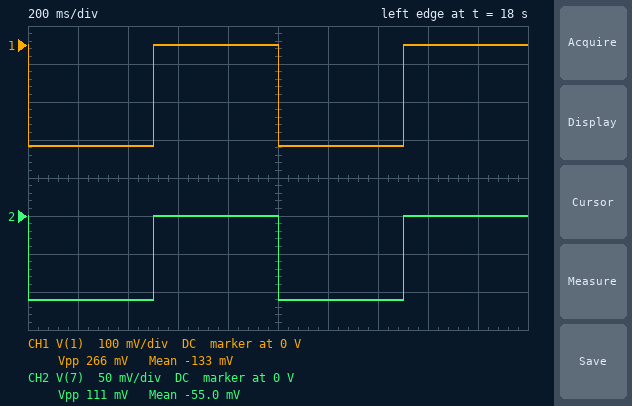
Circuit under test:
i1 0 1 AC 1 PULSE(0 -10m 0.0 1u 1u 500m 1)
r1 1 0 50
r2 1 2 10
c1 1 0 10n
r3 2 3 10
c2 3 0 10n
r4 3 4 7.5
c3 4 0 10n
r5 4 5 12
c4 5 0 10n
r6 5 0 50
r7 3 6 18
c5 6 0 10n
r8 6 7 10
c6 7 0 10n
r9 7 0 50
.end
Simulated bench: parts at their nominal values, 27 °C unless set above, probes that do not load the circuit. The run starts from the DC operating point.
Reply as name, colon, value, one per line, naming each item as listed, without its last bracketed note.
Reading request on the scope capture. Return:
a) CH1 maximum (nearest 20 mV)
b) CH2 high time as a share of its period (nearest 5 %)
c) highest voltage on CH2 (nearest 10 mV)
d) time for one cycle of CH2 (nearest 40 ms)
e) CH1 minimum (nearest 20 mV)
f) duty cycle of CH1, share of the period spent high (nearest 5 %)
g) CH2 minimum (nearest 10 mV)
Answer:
CH1 maximum: 0 V
CH2 high time as a share of its period: 50 %
highest voltage on CH2: 0 V
time for one cycle of CH2: 1.00 s
CH1 minimum: -260 mV
duty cycle of CH1, share of the period spent high: 50 %
CH2 minimum: -110 mV
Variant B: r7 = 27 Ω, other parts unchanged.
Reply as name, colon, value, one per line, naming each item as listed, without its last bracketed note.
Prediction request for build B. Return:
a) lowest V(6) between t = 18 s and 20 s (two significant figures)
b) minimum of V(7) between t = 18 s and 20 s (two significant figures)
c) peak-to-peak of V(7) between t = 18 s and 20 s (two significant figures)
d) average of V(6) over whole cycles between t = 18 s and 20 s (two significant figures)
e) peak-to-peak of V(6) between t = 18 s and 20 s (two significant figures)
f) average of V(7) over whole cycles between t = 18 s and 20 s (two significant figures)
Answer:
lowest V(6) between t = 18 s and 20 s: -120 mV
minimum of V(7) between t = 18 s and 20 s: -100 mV
peak-to-peak of V(7) between t = 18 s and 20 s: 100 mV
average of V(6) over whole cycles between t = 18 s and 20 s: -61 mV
peak-to-peak of V(6) between t = 18 s and 20 s: 120 mV
average of V(7) over whole cycles between t = 18 s and 20 s: -51 mV
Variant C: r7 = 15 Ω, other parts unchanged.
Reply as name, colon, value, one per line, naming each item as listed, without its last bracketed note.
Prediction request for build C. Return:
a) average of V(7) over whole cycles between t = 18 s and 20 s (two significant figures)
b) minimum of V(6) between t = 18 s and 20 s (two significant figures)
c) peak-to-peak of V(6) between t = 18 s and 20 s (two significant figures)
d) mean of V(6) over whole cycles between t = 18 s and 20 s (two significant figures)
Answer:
average of V(7) over whole cycles between t = 18 s and 20 s: -57 mV
minimum of V(6) between t = 18 s and 20 s: -140 mV
peak-to-peak of V(6) between t = 18 s and 20 s: 140 mV
mean of V(6) over whole cycles between t = 18 s and 20 s: -68 mV
